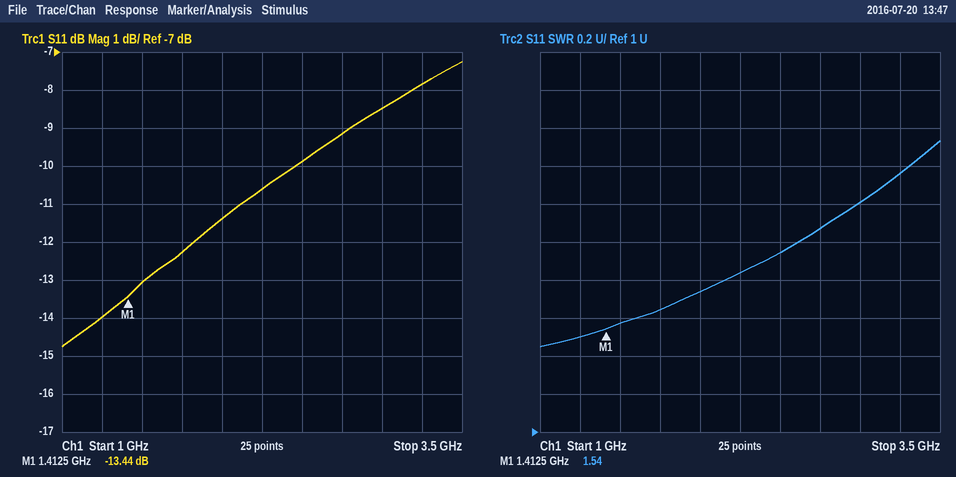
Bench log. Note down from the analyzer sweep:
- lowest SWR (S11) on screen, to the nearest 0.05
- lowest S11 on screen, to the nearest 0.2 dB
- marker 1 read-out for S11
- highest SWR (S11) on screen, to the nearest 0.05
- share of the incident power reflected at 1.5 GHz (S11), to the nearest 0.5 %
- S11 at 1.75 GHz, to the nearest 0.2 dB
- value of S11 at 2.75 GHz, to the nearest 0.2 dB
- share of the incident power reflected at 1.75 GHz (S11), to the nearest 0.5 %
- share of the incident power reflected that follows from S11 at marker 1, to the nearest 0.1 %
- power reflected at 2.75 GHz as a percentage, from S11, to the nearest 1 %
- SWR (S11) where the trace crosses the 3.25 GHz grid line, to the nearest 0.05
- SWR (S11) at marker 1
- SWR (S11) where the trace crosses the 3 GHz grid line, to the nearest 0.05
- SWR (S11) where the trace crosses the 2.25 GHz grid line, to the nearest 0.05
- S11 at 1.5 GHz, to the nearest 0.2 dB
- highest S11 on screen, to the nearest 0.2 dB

1.45
-14.8 dB
-13.44 dB
2.55
5.0 %
-12.2 dB
-9.2 dB
6.0 %
4.5 %
12 %
2.35
1.54
2.20
1.85
-13.0 dB
-7.2 dB
